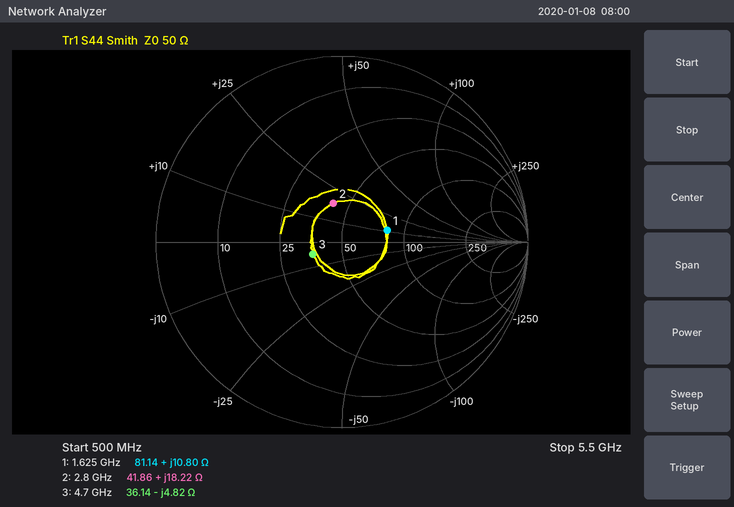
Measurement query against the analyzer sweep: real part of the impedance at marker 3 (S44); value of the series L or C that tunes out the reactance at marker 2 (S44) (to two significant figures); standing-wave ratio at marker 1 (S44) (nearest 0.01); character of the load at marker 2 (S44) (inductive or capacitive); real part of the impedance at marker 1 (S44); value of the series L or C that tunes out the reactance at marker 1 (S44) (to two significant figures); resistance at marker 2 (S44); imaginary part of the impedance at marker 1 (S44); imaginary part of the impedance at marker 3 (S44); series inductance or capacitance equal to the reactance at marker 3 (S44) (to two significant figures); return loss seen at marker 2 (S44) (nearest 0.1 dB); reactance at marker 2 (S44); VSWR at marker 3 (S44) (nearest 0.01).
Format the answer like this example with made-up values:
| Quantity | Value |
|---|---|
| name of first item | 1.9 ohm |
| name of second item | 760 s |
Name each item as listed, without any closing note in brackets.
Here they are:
| Quantity | Value |
|---|---|
| real part of the impedance at marker 3 | 36.14 Ω |
| value of the series L or C that tunes out the reactance at marker 2 (S44) | 3.1 pF |
| standing-wave ratio at marker 1 (S44) | 1.67 |
| character of the load at marker 2 (S44) | inductive |
| real part of the impedance at marker 1 | 81.14 Ω |
| value of the series L or C that tunes out the reactance at marker 1 (S44) | 9.1 pF |
| resistance at marker 2 | 41.86 Ω |
| imaginary part of the impedance at marker 1 | +10.80 Ω |
| imaginary part of the impedance at marker 3 | -4.82 Ω |
| series inductance or capacitance equal to the reactance at marker 3 (S44) | 7.0 pF |
| return loss seen at marker 2 (S44) | 13.4 dB |
| reactance at marker 2 | +18.22 Ω |
| VSWR at marker 3 (S44) | 1.41 |
